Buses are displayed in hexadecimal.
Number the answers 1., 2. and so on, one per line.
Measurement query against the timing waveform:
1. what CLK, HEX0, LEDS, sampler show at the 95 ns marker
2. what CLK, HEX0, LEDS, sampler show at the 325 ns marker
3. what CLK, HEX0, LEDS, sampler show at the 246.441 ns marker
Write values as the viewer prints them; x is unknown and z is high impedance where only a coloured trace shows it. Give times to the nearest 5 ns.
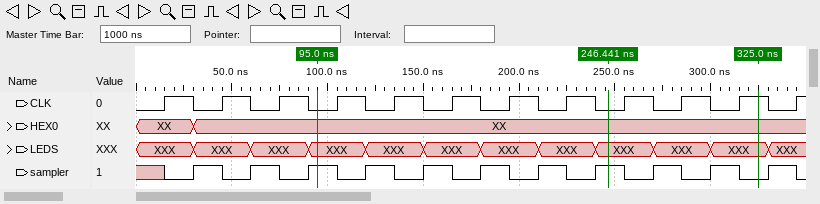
1. CLK=0, HEX0=XX, LEDS=XXX, sampler=1
2. CLK=1, HEX0=XX, LEDS=XXX, sampler=0
3. CLK=0, HEX0=XX, LEDS=XXX, sampler=1
